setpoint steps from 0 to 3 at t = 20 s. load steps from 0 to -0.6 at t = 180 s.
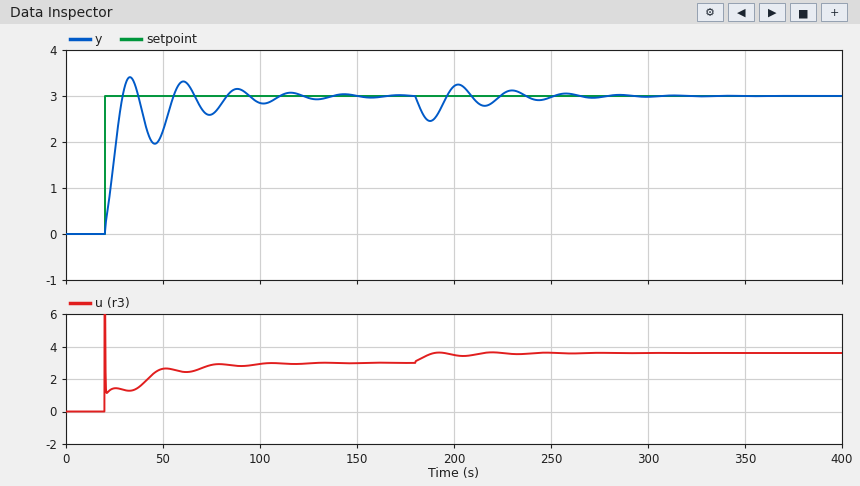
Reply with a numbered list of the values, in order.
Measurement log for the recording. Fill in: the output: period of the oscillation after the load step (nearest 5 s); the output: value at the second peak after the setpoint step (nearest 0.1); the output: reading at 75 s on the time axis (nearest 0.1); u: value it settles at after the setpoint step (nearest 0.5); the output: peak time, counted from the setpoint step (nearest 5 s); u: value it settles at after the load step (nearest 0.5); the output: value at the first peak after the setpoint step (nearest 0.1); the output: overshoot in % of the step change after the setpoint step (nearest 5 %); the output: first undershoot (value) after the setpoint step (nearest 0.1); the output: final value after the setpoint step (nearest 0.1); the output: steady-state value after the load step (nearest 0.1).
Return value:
1. 30 s
2. 3.3
3. 2.6
4. 3.0
5. 15 s
6. 3.5
7. 3.4
8. 15 %
9. 2.0
10. 3.0
11. 3.0
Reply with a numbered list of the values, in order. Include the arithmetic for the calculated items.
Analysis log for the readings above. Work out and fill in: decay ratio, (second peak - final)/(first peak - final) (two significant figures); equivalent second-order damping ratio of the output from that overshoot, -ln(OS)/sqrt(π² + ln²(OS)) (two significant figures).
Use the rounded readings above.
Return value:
1. (3.3 - 3) / (3.4 - 3) = 0.75
2. ln(0.15) = -1.897; 1.897 / sqrt(9.870 + 3.599) = 0.52
